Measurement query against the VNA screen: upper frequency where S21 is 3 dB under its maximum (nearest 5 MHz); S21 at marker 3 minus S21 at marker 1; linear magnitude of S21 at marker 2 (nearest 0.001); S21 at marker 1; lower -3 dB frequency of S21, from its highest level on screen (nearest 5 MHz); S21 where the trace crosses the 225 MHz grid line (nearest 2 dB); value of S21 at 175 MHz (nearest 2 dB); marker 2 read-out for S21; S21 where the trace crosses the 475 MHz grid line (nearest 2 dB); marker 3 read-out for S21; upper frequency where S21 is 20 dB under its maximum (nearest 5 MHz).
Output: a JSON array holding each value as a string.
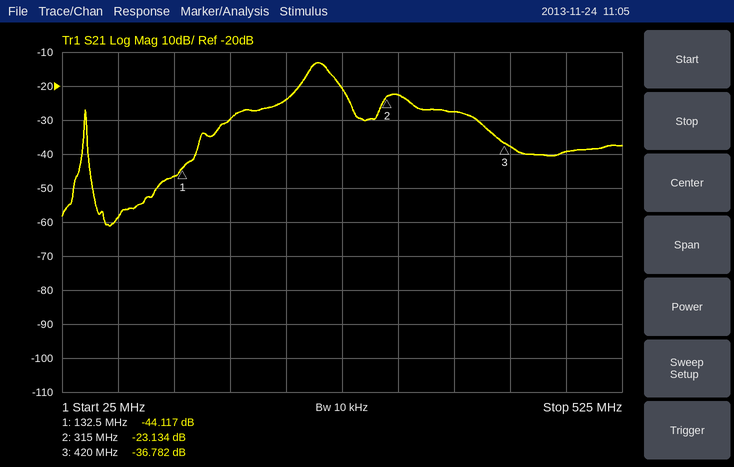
["265 MHz", "7.335 dB", "0.070", "-44.117 dB", "245 MHz", "-24 dB", "-30 dB", "-23.134 dB", "-40 dB", "-36.782 dB", "405 MHz"]
